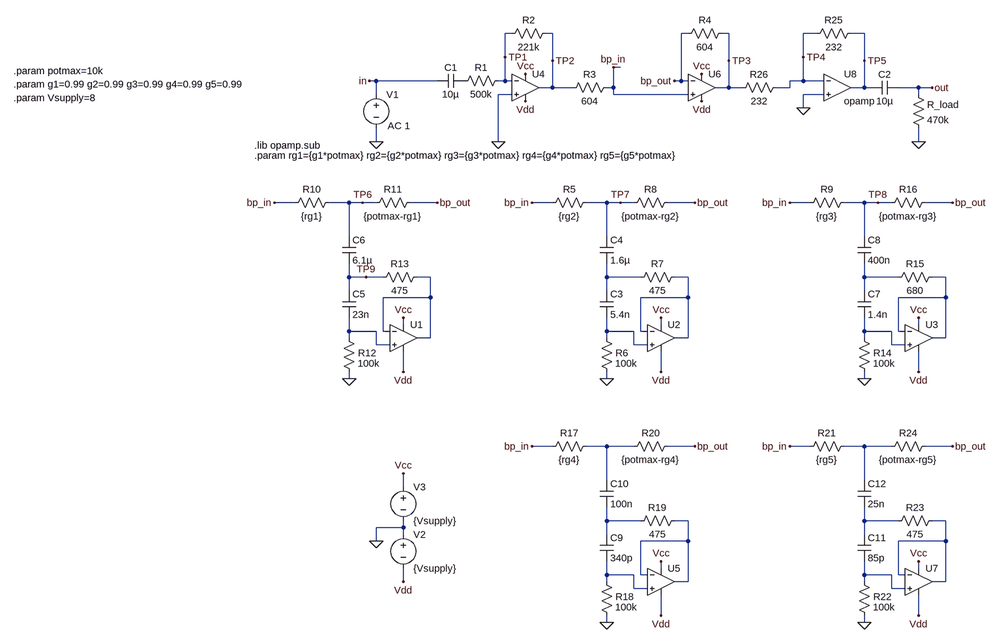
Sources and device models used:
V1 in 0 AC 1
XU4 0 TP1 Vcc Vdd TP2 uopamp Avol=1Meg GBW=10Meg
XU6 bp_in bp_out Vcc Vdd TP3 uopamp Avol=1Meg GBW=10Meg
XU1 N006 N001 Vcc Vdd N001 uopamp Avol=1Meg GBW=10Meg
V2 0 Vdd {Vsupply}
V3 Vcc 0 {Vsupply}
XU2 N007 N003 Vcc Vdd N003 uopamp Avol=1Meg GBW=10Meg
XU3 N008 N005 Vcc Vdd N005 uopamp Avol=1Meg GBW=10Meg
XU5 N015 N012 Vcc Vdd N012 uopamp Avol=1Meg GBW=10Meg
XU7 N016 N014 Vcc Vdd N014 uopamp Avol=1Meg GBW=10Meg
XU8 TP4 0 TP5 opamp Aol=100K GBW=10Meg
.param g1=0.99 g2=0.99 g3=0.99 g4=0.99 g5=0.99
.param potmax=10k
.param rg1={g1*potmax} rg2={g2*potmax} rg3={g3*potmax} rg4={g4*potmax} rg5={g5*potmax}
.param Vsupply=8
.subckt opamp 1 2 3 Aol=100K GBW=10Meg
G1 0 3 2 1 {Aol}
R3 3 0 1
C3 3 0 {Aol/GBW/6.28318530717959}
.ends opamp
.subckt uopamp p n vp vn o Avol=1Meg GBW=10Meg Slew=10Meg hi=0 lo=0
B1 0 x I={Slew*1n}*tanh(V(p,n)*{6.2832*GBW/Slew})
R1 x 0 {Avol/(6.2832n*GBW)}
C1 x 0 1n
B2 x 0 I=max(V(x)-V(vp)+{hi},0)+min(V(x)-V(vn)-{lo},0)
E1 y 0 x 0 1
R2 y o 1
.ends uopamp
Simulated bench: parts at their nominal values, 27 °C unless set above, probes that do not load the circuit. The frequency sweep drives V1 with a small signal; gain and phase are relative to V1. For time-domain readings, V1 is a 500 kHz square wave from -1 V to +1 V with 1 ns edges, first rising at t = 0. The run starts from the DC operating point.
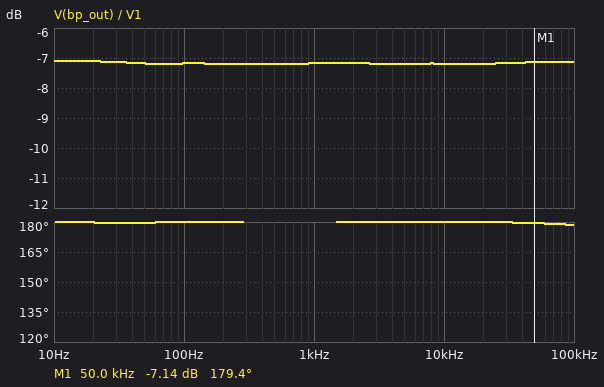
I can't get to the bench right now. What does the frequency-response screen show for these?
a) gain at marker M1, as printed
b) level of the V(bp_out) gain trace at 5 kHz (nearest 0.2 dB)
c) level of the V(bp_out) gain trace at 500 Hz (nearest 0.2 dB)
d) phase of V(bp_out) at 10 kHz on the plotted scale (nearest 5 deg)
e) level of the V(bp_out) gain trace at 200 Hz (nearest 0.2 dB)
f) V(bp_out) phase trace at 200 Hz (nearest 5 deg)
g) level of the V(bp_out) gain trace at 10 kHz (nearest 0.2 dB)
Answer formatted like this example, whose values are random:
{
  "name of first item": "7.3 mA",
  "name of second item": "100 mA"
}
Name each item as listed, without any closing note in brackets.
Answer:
{
  "gain at marker M1, as printed": "-7.14 dB",
  "level of the V(bp_out) gain trace at 5 kHz": "-7.2 dB",
  "level of the V(bp_out) gain trace at 500 Hz": "-7.2 dB",
  "phase of V(bp_out) at 10 kHz on the plotted scale": "180 deg",
  "level of the V(bp_out) gain trace at 200 Hz": "-7.2 dB",
  "V(bp_out) phase trace at 200 Hz": "180 deg",
  "level of the V(bp_out) gain trace at 10 kHz": "-7.2 dB"
}
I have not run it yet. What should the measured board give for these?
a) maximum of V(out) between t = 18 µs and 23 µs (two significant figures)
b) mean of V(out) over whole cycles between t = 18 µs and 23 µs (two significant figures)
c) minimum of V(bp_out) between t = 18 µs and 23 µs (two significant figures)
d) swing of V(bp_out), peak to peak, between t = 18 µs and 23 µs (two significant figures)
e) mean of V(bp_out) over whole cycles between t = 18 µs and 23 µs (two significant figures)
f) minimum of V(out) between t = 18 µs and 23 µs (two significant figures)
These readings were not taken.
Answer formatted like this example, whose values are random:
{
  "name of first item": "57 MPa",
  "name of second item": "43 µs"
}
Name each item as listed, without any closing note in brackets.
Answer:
{
  "maximum of V(out) between t = 18 µs and 23 µs": "1.8 V",
  "mean of V(out) over whole cycles between t = 18 µs and 23 µs": "960 mV",
  "minimum of V(bp_out) between t = 18 µs and 23 µs": "-1.0 V",
  "swing of V(bp_out), peak to peak, between t = 18 µs and 23 µs": "1.1 V",
  "mean of V(bp_out) over whole cycles between t = 18 µs and 23 µs": "-440 mV",
  "minimum of V(out) between t = 18 µs and 23 µs": "110 mV"
}
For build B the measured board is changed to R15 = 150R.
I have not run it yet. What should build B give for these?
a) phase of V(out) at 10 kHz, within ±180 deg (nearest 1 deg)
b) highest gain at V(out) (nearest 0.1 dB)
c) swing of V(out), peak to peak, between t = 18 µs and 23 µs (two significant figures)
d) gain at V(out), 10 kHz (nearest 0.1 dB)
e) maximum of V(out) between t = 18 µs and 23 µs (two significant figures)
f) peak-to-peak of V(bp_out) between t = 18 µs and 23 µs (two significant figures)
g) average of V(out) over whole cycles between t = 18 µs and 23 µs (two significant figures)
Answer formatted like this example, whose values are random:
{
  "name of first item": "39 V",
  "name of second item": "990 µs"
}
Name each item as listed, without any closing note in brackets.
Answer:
{
  "phase of V(out) at 10 kHz, within ±180 deg": "-13 deg",
  "highest gain at V(out)": "4.5 dB",
  "swing of V(out), peak to peak, between t = 18 µs and 23 µs": "2.1 V",
  "gain at V(out), 10 kHz": "-0.3 dB",
  "maximum of V(out) between t = 18 µs and 23 µs": "2.2 V",
  "peak-to-peak of V(bp_out) between t = 18 µs and 23 µs": "1.2 V",
  "average of V(out) over whole cycles between t = 18 µs and 23 µs": "1.1 V"
}
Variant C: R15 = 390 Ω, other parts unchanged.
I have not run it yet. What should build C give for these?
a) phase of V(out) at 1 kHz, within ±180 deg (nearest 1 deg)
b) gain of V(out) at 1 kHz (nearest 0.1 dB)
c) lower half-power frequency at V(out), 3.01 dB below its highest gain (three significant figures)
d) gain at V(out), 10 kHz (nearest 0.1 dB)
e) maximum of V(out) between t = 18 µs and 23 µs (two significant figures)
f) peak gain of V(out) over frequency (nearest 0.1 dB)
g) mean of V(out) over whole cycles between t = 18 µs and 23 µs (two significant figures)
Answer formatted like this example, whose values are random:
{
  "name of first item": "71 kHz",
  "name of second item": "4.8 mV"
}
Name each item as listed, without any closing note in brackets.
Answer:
{
  "phase of V(out) at 1 kHz, within ±180 deg": "3 deg",
  "gain of V(out) at 1 kHz": "0.7 dB",
  "lower half-power frequency at V(out), 3.01 dB below its highest gain": "33.4 Hz",
  "gain at V(out), 10 kHz": "-0.7 dB",
  "maximum of V(out) between t = 18 µs and 23 µs": "1.9 V",
  "peak gain of V(out) over frequency": "0.8 dB",
  "mean of V(out) over whole cycles between t = 18 µs and 23 µs": "1.0 V"
}
